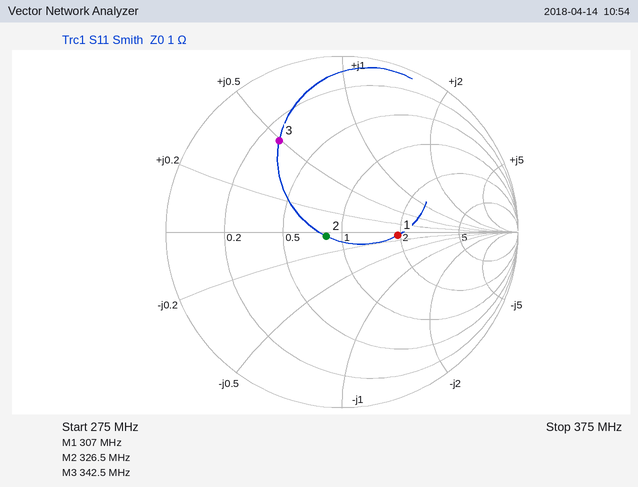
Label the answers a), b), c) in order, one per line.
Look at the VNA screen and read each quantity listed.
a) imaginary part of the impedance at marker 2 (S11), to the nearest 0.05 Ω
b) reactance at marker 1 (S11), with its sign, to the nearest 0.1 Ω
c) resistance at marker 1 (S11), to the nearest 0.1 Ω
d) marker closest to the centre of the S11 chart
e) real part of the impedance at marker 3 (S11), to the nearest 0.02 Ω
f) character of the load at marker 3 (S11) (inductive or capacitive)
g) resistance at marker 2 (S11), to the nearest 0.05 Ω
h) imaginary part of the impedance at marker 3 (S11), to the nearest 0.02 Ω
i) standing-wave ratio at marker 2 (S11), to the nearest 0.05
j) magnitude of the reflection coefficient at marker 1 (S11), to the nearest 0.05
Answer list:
a) -0.05 Ω
b) -0.1 Ω
c) 1.9 Ω
d) marker 2
e) 0.28 Ω
f) inductive
g) 0.85 Ω
h) +0.50 Ω
i) 1.20
j) 0.30
